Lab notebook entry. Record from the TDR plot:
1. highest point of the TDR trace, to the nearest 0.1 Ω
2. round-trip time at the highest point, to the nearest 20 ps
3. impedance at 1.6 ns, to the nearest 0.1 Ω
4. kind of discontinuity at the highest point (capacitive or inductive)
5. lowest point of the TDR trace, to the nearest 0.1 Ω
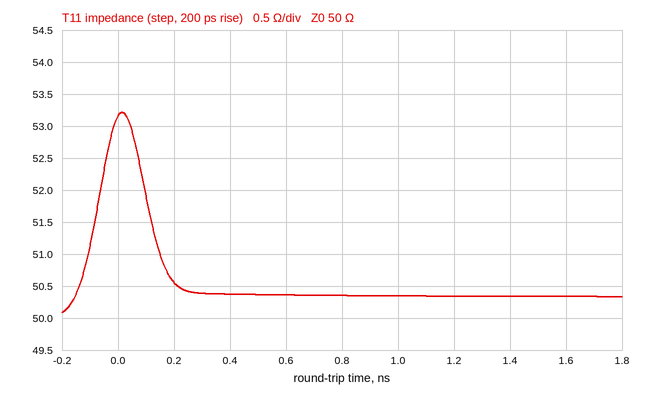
53.2 Ω
20 ps
50.3 Ω
inductive
50.1 Ω
